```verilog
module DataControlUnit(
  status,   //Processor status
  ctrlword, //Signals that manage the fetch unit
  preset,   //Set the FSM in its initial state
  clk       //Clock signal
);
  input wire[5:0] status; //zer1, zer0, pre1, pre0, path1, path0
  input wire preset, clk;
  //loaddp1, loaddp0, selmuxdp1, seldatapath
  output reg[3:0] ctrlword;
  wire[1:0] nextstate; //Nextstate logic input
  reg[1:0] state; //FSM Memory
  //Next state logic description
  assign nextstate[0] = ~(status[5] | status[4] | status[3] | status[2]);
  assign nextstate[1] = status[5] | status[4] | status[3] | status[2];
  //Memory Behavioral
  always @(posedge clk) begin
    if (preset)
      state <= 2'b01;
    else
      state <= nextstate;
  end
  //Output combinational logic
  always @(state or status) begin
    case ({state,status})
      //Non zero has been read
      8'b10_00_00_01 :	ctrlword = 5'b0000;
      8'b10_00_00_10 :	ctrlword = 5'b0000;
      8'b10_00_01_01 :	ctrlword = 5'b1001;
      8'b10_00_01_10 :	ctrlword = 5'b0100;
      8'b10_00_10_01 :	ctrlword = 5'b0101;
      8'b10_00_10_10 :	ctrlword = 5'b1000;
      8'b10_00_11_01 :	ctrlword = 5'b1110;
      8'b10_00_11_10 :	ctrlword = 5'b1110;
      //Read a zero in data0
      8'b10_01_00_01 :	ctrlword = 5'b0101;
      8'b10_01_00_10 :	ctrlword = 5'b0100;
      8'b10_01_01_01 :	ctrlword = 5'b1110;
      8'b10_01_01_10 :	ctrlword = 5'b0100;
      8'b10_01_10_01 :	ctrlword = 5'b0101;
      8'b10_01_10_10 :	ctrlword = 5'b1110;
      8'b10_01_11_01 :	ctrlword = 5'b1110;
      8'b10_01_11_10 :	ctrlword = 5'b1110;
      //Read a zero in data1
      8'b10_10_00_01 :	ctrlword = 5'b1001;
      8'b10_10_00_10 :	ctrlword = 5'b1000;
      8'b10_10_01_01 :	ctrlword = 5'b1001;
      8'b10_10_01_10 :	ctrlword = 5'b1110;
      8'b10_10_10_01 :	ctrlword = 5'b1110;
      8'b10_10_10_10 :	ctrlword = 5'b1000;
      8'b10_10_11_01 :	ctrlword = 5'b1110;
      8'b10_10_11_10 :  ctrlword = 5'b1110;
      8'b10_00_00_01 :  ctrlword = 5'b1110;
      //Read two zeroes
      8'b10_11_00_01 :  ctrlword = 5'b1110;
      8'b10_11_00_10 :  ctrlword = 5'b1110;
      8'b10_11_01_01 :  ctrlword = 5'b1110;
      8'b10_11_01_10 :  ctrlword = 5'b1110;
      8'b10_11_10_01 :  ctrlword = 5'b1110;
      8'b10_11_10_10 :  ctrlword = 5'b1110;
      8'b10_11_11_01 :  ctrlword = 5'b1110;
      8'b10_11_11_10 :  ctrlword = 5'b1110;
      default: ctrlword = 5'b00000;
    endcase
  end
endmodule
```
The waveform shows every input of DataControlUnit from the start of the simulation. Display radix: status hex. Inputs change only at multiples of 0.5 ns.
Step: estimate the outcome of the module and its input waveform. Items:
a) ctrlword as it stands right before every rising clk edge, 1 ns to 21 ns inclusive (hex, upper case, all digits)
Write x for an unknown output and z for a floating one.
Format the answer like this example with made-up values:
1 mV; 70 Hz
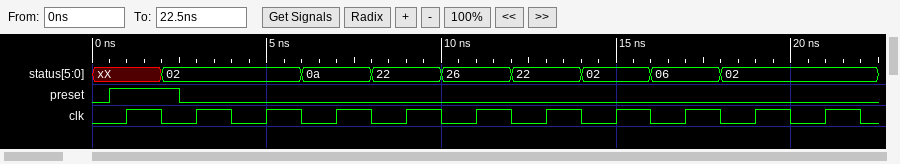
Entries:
0, 0, 0, 0, 8, E, 8, 0, 0, 0, 0
